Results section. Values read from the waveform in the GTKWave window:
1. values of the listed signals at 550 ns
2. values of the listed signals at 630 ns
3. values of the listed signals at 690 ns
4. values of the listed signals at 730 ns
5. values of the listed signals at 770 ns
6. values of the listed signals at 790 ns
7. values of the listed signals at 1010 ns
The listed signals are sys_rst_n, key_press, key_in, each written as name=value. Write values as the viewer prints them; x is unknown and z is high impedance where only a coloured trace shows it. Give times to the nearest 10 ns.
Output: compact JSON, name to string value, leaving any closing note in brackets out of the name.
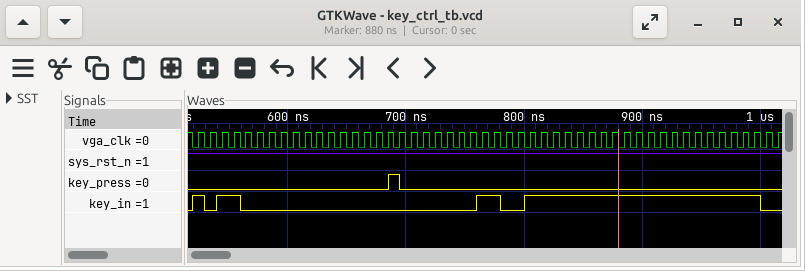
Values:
{"values of the listed signals at 550 ns": "sys_rst_n=1, key_press=0, key_in=1", "values of the listed signals at 630 ns": "sys_rst_n=1, key_press=0, key_in=0", "values of the listed signals at 690 ns": "sys_rst_n=1, key_press=1, key_in=0", "values of the listed signals at 730 ns": "sys_rst_n=1, key_press=0, key_in=0", "values of the listed signals at 770 ns": "sys_rst_n=1, key_press=0, key_in=1", "values of the listed signals at 790 ns": "sys_rst_n=1, key_press=0, key_in=0", "values of the listed signals at 1010 ns": "sys_rst_n=1, key_press=0, key_in=0"}
